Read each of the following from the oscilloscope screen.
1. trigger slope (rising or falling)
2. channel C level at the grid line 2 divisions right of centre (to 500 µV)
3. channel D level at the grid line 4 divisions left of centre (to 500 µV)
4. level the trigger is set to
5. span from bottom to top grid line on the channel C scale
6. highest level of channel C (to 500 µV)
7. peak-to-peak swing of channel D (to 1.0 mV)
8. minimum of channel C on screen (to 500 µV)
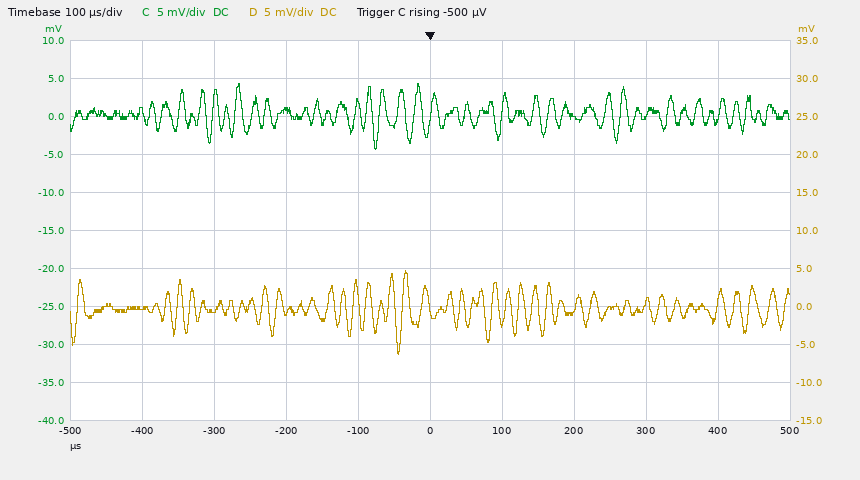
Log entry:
rising
0.0 mV
0.0 mV
-500 µV
50 mV
4.5 mV
11.0 mV
-4.5 mV
